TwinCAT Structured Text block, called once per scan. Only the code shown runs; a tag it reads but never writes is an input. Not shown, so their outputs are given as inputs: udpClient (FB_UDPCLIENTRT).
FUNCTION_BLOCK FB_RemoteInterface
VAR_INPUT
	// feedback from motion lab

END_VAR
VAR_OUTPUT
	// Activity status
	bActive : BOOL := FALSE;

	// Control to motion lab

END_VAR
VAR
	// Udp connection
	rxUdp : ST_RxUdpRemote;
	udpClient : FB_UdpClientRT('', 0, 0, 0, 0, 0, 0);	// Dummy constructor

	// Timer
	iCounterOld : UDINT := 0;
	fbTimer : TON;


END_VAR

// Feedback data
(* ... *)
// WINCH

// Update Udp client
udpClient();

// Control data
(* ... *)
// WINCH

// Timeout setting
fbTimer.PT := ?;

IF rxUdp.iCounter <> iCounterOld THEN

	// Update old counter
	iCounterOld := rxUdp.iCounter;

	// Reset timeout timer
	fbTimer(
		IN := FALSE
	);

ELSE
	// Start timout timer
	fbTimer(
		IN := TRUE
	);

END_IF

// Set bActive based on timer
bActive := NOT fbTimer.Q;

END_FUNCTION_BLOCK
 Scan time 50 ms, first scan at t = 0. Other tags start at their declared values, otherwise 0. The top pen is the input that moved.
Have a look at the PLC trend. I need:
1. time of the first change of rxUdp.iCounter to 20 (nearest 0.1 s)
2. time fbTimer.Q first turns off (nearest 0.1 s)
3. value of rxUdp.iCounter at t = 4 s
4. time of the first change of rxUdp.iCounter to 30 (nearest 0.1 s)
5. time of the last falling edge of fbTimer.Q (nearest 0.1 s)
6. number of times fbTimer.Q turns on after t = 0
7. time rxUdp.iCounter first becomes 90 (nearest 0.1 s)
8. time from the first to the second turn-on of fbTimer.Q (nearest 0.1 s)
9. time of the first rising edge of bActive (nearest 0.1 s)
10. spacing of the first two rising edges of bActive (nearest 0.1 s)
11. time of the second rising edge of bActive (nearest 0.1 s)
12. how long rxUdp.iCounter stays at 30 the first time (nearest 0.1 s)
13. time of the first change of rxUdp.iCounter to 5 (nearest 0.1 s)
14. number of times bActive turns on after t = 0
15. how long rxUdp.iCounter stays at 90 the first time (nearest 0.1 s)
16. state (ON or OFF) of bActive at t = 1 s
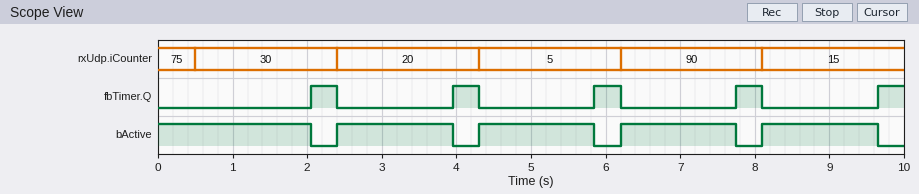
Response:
2.4 s
2.4 s
20
0.5 s
8.1 s
5
6.2 s
1.9 s
2.4 s
1.9 s
4.3 s
1.9 s
4.3 s
4
1.9 s
ON
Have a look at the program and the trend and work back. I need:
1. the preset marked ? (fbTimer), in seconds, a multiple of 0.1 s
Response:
1.5 s
